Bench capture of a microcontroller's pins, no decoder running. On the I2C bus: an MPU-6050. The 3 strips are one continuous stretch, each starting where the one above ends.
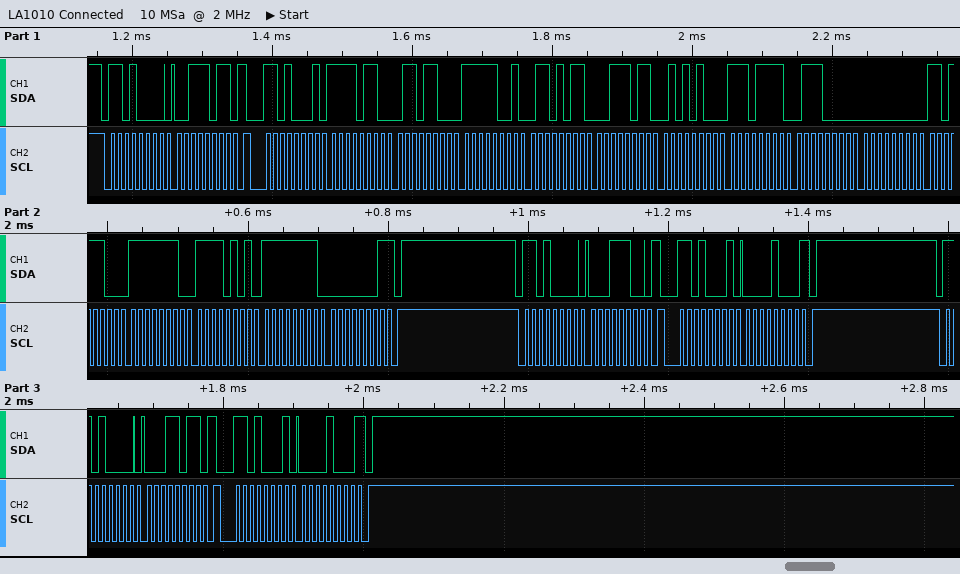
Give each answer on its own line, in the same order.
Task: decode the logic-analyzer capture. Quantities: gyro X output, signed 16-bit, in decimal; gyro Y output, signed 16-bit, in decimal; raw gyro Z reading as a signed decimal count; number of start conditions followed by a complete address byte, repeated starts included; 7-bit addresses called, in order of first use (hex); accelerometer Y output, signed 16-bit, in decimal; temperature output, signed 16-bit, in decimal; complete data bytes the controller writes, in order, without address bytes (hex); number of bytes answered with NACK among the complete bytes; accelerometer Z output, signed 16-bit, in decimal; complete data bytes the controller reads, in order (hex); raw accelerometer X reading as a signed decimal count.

220
-267
-255
6
0x68
-1685
-4240
3B 1C 1B
3
15188
F6 6C F9 6B 3B 54 EF 70 00 DC FE F5 FF 01 08 08
-2452
